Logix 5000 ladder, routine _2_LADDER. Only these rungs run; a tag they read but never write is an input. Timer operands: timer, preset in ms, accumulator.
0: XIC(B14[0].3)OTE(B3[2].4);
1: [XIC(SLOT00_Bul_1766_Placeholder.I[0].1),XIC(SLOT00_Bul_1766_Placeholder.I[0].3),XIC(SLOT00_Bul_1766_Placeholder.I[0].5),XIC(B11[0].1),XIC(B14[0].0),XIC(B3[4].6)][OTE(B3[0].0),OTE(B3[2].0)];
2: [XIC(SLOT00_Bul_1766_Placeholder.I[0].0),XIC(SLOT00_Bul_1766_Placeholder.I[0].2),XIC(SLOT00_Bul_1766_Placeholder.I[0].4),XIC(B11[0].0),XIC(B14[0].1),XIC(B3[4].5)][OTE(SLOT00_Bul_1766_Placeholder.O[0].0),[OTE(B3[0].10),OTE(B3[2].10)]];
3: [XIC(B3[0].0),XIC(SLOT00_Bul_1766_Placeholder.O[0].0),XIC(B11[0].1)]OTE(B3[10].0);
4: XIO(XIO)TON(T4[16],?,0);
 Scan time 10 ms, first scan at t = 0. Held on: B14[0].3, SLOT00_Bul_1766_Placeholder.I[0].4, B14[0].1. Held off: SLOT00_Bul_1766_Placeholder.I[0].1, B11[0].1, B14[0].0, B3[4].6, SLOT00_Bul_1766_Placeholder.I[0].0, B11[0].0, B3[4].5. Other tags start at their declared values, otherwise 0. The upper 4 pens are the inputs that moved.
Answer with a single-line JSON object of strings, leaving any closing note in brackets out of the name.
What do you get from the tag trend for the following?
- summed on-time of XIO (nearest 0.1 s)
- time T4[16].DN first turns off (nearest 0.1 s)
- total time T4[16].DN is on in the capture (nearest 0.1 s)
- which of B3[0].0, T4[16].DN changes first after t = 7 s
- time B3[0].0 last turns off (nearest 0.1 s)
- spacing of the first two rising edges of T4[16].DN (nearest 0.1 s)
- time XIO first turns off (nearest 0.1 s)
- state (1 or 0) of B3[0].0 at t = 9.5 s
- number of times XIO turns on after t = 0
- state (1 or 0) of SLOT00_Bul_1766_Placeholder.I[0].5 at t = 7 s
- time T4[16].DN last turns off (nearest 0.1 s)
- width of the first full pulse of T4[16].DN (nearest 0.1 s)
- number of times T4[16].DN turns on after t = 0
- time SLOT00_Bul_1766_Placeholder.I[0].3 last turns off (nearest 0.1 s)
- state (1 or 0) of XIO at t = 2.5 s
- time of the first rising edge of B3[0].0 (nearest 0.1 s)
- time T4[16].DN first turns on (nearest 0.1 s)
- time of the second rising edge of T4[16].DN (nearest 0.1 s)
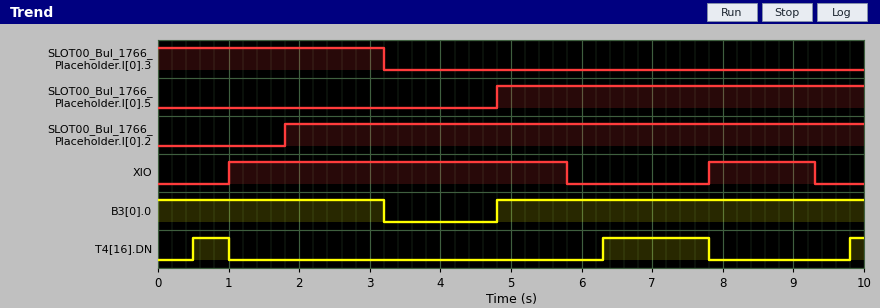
{"summed on-time of XIO": "6.3 s", "time T4[16].DN first turns off": "1.0 s", "total time T4[16].DN is on in the capture": "2.2 s", "which of B3[0].0, T4[16].DN changes first after t = 7 s": "T4[16].DN", "time B3[0].0 last turns off": "3.2 s", "spacing of the first two rising edges of T4[16].DN": "5.8 s", "time XIO first turns off": "5.8 s", "state (1 or 0) of B3[0].0 at t = 9.5 s": "1", "number of times XIO turns on after t = 0": "2", "state (1 or 0) of SLOT00_Bul_1766_Placeholder.I[0].5 at t = 7 s": "1", "time T4[16].DN last turns off": "7.8 s", "width of the first full pulse of T4[16].DN": "0.5 s", "number of times T4[16].DN turns on after t = 0": "3", "time SLOT00_Bul_1766_Placeholder.I[0].3 last turns off": "3.2 s", "state (1 or 0) of XIO at t = 2.5 s": "1", "time of the first rising edge of B3[0].0": "4.8 s", "time T4[16].DN first turns on": "0.5 s", "time of the second rising edge of T4[16].DN": "6.3 s"}
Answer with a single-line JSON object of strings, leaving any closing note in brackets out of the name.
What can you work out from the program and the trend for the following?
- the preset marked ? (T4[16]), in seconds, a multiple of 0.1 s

{"the preset marked ? (T4[16]), in seconds, a multiple of 0.1 s": "0.5 s"}
